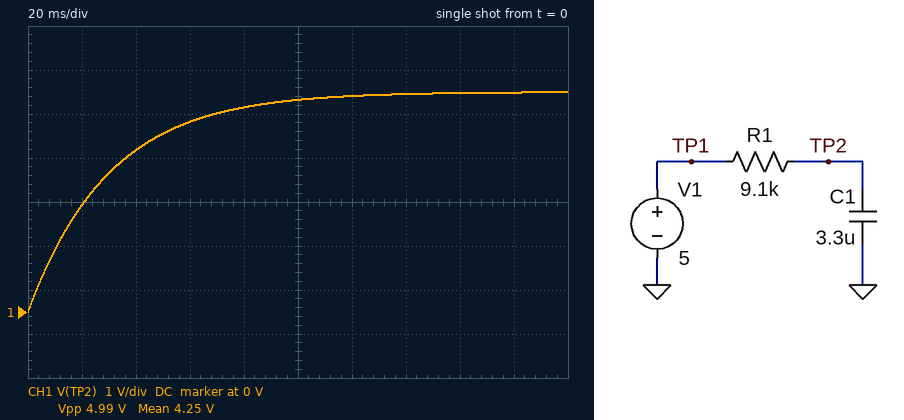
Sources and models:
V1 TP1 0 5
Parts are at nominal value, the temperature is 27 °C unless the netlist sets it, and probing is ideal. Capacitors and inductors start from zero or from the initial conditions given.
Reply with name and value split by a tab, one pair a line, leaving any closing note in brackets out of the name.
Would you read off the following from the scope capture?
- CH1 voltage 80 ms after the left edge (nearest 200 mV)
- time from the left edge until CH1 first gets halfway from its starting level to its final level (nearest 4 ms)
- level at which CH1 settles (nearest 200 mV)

CH1 voltage 80 ms after the left edge	4.6 V
time from the left edge until CH1 first gets halfway from its starting level to its final level	20 ms
level at which CH1 settles	5.0 V
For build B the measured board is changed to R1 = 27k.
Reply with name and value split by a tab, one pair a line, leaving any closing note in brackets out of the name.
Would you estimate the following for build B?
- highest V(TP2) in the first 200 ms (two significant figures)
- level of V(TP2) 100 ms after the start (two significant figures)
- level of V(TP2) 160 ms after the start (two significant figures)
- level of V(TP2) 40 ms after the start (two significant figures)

highest V(TP2) in the first 200 ms	4.5 V
level of V(TP2) 100 ms after the start	3.4 V
level of V(TP2) 160 ms after the start	4.2 V
level of V(TP2) 40 ms after the start	1.8 V
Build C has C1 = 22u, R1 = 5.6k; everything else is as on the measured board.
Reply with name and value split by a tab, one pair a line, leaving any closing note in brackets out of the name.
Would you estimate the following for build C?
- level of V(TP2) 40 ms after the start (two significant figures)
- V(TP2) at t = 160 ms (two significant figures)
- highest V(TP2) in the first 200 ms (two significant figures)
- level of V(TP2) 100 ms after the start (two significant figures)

level of V(TP2) 40 ms after the start	1.4 V
V(TP2) at t = 160 ms	3.6 V
highest V(TP2) in the first 200 ms	4.0 V
level of V(TP2) 100 ms after the start	2.8 V
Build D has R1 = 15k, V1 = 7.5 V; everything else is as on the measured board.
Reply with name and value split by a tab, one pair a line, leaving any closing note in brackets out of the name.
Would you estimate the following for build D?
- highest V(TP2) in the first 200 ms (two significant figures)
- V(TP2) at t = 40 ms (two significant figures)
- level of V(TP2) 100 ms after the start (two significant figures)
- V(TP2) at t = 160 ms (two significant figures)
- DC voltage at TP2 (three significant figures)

highest V(TP2) in the first 200 ms	7.4 V
V(TP2) at t = 40 ms	4.2 V
level of V(TP2) 100 ms after the start	6.5 V
V(TP2) at t = 160 ms	7.2 V
DC voltage at TP2	7.50 V
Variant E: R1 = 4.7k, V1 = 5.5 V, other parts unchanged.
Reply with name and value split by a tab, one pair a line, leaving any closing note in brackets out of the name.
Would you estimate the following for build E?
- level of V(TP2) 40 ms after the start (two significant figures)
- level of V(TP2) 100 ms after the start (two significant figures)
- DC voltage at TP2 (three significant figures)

level of V(TP2) 40 ms after the start	5.1 V
level of V(TP2) 100 ms after the start	5.5 V
DC voltage at TP2	5.50 V
